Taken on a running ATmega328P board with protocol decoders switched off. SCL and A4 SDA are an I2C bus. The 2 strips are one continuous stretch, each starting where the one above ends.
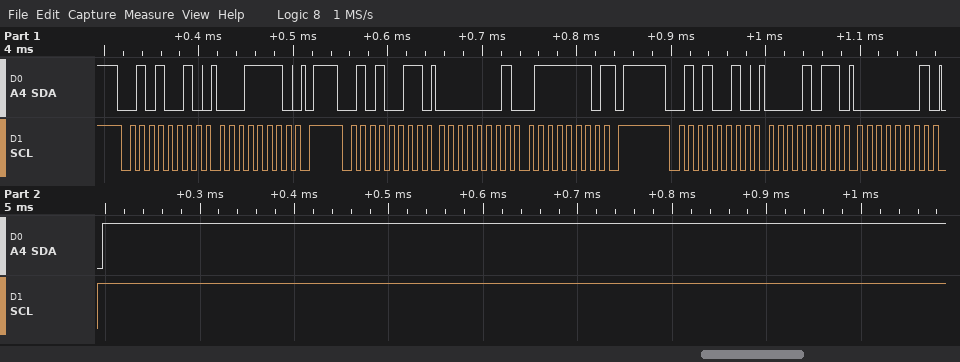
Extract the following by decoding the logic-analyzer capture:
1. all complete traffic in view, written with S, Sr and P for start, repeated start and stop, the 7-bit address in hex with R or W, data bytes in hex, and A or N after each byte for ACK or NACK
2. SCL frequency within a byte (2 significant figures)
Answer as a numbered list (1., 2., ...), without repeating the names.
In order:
1. S 29W A 1E A P S 29R A 01 A 7E N P S 29W A 0B A 01 A P
2. 100 kHz
